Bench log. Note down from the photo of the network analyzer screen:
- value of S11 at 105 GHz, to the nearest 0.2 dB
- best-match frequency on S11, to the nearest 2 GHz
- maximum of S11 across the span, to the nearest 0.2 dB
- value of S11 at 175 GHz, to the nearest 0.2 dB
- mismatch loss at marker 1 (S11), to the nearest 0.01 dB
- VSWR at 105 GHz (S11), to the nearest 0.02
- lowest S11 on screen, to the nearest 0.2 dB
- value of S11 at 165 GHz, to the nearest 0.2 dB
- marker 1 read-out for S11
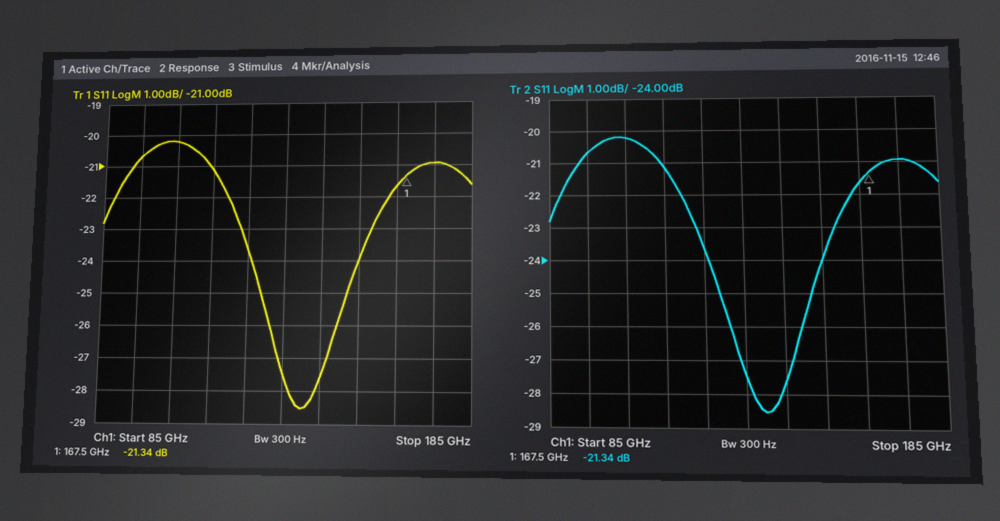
-20.2 dB
140 GHz
-20.2 dB
-21.0 dB
0.03 dB
1.22
-28.6 dB
-21.6 dB
-21.34 dB
